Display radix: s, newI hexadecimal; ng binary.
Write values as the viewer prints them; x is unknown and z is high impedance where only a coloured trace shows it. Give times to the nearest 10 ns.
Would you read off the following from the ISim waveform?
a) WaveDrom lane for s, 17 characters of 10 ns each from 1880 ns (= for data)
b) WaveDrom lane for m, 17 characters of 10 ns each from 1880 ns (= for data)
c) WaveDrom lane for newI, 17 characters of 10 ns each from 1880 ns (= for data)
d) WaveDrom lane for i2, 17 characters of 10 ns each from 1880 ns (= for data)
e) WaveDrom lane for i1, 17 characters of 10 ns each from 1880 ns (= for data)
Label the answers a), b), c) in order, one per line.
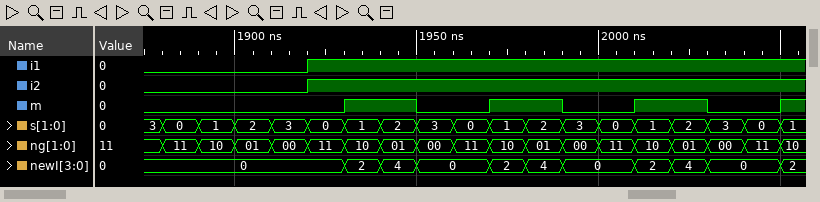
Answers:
a) {name: 's', wave: '=================', data: '0 1 2 3 0 1 2 3 0 1 2 3 0 1 2 3 0'}
b) {name: 'm', wave: '0....1.0.1.0.1.0.'}
c) {name: 'newI', wave: '=....===.===.===.', data: '0 2 4 0 2 4 0 2 4 0'}
d) {name: 'i2', wave: '0...1............'}
e) {name: 'i1', wave: '0...1............'}
